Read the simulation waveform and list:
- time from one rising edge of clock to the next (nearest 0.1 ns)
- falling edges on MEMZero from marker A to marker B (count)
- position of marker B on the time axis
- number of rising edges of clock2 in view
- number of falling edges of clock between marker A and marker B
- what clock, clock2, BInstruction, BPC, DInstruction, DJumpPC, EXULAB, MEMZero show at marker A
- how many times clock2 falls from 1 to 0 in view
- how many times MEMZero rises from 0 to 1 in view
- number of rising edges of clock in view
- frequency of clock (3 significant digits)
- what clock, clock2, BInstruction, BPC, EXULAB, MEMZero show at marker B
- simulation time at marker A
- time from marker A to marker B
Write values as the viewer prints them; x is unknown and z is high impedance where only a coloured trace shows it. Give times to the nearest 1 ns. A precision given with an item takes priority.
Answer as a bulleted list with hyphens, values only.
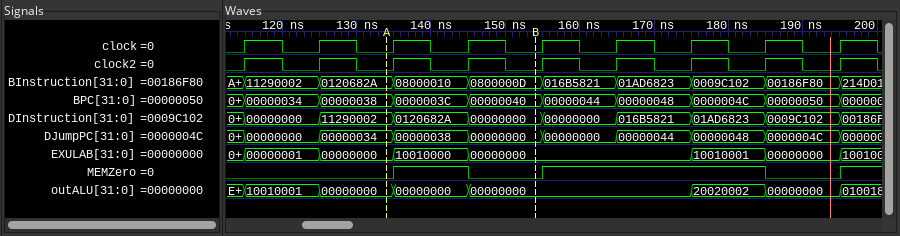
- 10 ns
- 1
- 154 ns
- 9
- 2
- clock=0, clock2=0, BInstruction=0120682A, BPC=00000038, DInstruction=11290002, DJumpPC=00000034, EXULAB=00000000, MEMZero=0
- 9
- 3
- 9
- 100 MHz
- clock=0, clock2=0, BInstruction=0800000D, BPC=00000040, EXULAB=00000000, MEMZero=0
- 134 ns
- 20 ns
